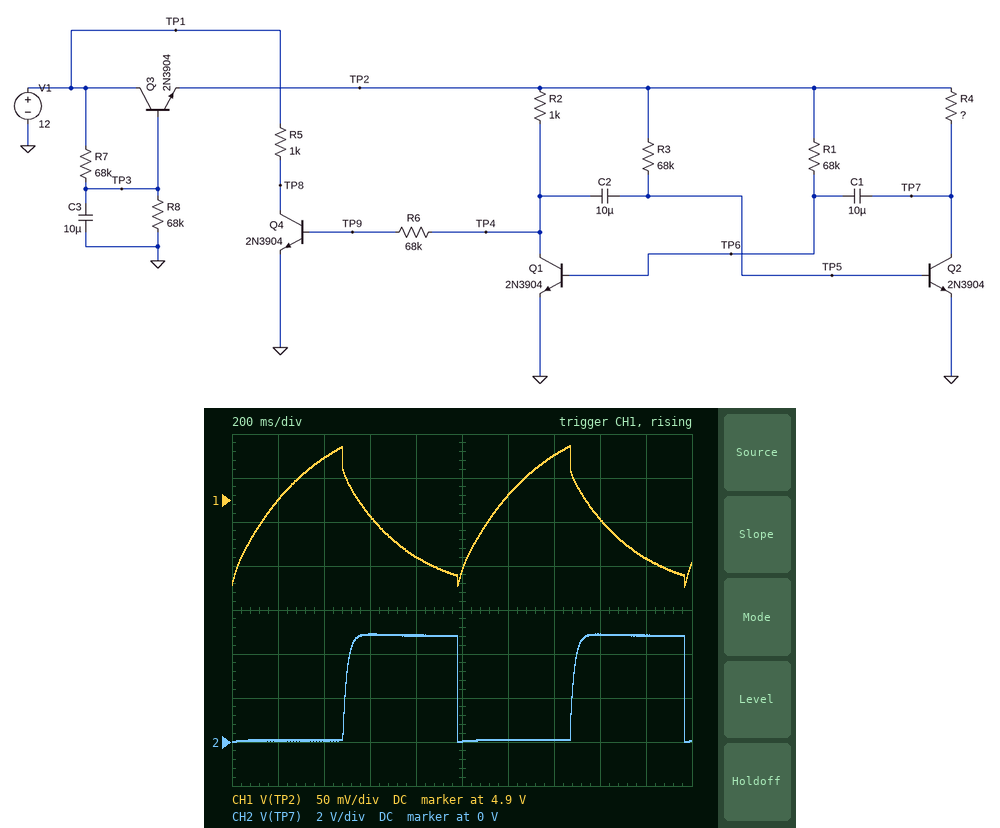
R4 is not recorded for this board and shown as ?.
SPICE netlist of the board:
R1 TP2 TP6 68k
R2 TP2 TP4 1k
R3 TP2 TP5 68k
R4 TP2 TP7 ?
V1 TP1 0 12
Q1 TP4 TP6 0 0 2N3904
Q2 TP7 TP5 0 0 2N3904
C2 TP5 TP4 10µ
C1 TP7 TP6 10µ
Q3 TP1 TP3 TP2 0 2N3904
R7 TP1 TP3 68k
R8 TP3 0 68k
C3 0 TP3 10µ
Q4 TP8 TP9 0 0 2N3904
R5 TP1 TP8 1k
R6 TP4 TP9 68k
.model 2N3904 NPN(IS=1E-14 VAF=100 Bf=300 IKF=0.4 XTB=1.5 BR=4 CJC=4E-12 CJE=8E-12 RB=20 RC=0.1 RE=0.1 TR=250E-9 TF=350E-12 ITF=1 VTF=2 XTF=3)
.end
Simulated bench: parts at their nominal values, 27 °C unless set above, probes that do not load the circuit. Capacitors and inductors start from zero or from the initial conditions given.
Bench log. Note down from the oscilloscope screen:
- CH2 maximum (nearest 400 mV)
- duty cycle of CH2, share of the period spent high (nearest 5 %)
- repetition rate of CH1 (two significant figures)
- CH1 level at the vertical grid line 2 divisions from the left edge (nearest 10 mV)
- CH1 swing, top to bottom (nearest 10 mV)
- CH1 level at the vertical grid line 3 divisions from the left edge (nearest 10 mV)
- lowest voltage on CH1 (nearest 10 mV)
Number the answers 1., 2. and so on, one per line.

1. 4.8 V
2. 50 %
3. 1.0 Hz
4. 4.95 V
5. 160 mV
6. 4.88 V
7. 4.80 V
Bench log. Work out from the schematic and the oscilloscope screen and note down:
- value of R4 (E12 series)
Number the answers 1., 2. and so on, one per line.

1. 1.8 kΩ
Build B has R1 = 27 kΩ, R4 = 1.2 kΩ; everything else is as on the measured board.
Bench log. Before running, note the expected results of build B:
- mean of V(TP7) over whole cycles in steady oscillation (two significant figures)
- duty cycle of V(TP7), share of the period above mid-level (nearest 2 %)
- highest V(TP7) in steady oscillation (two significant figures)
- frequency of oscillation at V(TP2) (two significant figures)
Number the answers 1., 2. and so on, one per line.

1. 3.4 V
2. 70 %
3. 4.8 V
4. 1.4 Hz
